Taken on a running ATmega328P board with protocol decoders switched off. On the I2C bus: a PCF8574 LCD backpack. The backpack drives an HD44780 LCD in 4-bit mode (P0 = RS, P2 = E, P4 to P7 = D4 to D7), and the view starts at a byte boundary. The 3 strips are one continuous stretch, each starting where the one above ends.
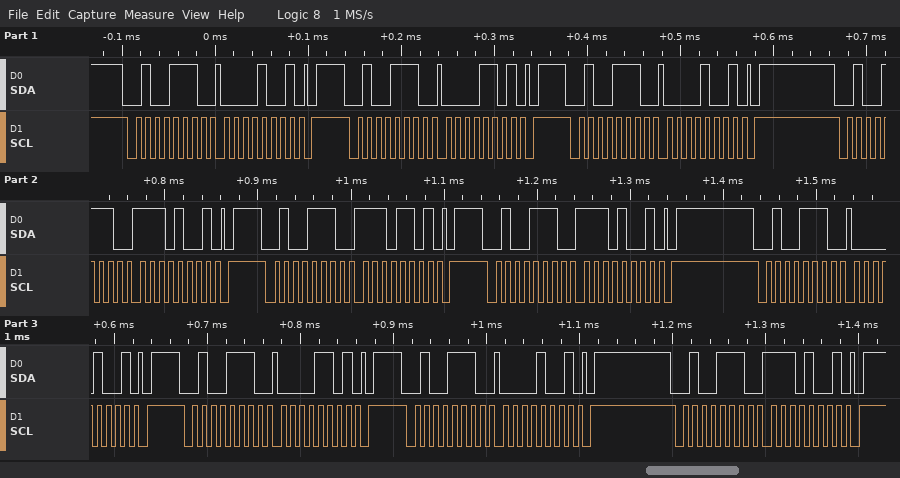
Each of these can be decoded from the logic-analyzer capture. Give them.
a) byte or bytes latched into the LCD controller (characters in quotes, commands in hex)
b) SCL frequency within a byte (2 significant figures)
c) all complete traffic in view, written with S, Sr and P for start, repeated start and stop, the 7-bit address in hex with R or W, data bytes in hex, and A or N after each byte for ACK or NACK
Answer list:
data 0x0E
100 kHz
S 27W A 09 A P S 27W A 0D A P S 27W A 09 A P S 27W A E9 A P S 27W A ED A P S 27W A E9 A P S 27W A 09 A P S 27W A 0D A P S 27W A 09 A P S 27W A E9 A P
